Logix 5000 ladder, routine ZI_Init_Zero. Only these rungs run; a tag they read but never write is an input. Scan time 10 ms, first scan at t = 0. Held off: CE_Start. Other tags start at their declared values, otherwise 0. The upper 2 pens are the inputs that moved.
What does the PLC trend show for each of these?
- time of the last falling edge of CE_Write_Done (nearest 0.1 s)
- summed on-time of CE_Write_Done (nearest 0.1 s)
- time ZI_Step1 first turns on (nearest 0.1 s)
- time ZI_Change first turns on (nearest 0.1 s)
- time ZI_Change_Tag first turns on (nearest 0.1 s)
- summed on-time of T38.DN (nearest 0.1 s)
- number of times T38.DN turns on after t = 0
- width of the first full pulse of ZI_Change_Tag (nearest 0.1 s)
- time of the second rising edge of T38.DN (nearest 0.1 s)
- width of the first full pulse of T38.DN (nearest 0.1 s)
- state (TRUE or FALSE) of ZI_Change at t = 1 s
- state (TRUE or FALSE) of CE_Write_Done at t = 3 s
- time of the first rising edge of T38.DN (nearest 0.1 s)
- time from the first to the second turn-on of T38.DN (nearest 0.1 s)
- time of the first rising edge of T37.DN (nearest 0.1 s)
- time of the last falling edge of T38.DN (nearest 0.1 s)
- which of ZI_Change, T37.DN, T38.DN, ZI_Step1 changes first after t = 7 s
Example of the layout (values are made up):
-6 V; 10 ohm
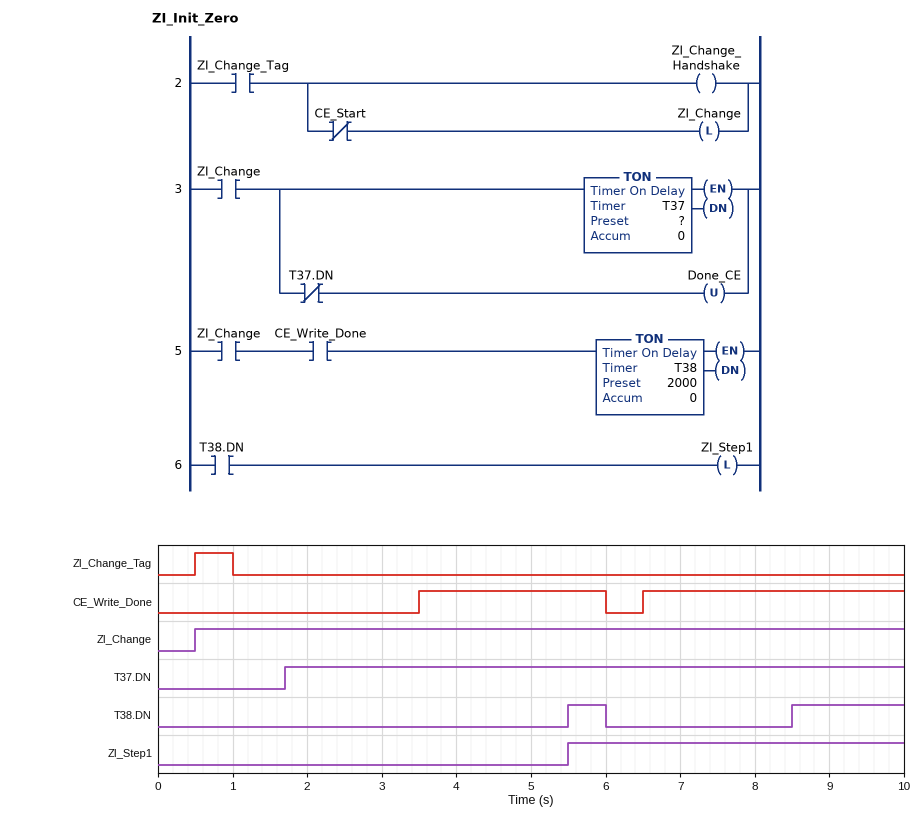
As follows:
6.0 s; 6.0 s; 5.5 s; 0.5 s; 0.5 s; 2.0 s; 2; 0.5 s; 8.5 s; 0.5 s; TRUE; FALSE; 5.5 s; 3.0 s; 1.7 s; 6.0 s; T38.DN
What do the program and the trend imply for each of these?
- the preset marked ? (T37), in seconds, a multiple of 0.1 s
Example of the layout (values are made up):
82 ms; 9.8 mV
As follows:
1.2 s
